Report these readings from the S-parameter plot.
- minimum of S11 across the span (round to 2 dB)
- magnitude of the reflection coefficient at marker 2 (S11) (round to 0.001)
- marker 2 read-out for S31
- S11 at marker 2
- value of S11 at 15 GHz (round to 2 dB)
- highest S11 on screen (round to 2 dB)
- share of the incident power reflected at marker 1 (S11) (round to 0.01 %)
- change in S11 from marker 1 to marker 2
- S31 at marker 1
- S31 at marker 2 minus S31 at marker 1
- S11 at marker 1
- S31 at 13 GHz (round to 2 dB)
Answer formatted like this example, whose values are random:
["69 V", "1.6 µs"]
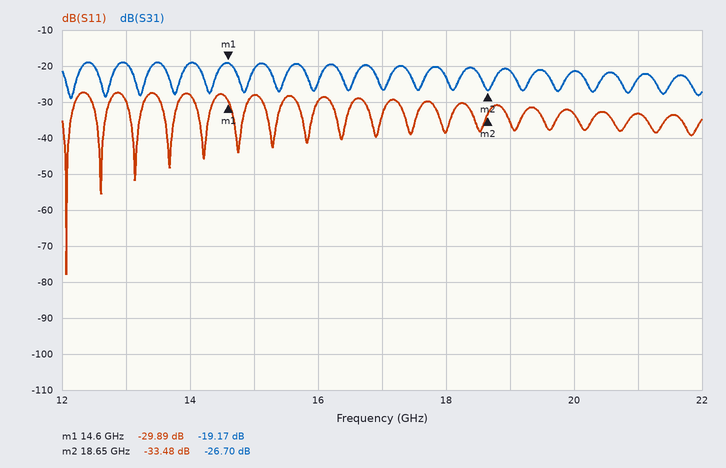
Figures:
["-78 dB", "0.021", "-26.70 dB", "-33.48 dB", "-28 dB", "-28 dB", "0.10 %", "-3.59 dB", "-19.17 dB", "-7.53 dB", "-29.89 dB", "-20 dB"]
